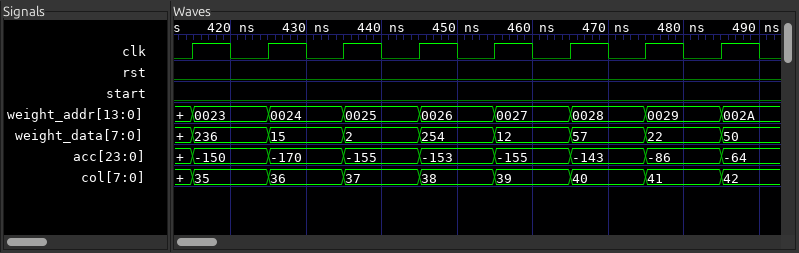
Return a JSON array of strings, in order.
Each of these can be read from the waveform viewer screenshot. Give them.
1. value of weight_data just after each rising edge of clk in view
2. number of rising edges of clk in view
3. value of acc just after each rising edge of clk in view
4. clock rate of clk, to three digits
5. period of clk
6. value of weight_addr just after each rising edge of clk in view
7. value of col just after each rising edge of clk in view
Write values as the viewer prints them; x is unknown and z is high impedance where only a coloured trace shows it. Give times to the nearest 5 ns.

["236, 15, 2, 254, 12, 57, 22, 50", "8", "-150, -170, -155, -153, -155, -143, -86, -64", "100 MHz", "10 ns", "0023, 0024, 0025, 0026, 0027, 0028, 0029, 002A", "35, 36, 37, 38, 39, 40, 41, 42"]
